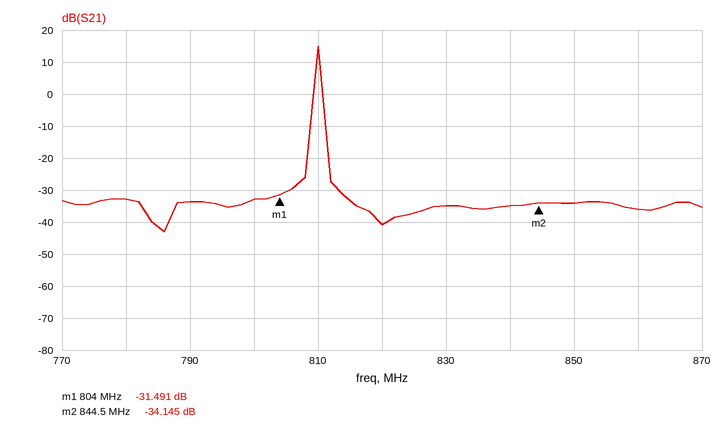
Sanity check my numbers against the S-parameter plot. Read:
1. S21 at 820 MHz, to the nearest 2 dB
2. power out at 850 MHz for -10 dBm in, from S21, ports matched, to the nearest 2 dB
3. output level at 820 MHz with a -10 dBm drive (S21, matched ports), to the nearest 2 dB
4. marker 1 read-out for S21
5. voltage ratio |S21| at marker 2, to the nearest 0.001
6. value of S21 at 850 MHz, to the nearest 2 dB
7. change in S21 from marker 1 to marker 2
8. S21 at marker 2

-40 dB
-44 dBm
-50 dBm
-31.491 dB
0.020
-34 dB
-2.654 dB
-34.145 dB
